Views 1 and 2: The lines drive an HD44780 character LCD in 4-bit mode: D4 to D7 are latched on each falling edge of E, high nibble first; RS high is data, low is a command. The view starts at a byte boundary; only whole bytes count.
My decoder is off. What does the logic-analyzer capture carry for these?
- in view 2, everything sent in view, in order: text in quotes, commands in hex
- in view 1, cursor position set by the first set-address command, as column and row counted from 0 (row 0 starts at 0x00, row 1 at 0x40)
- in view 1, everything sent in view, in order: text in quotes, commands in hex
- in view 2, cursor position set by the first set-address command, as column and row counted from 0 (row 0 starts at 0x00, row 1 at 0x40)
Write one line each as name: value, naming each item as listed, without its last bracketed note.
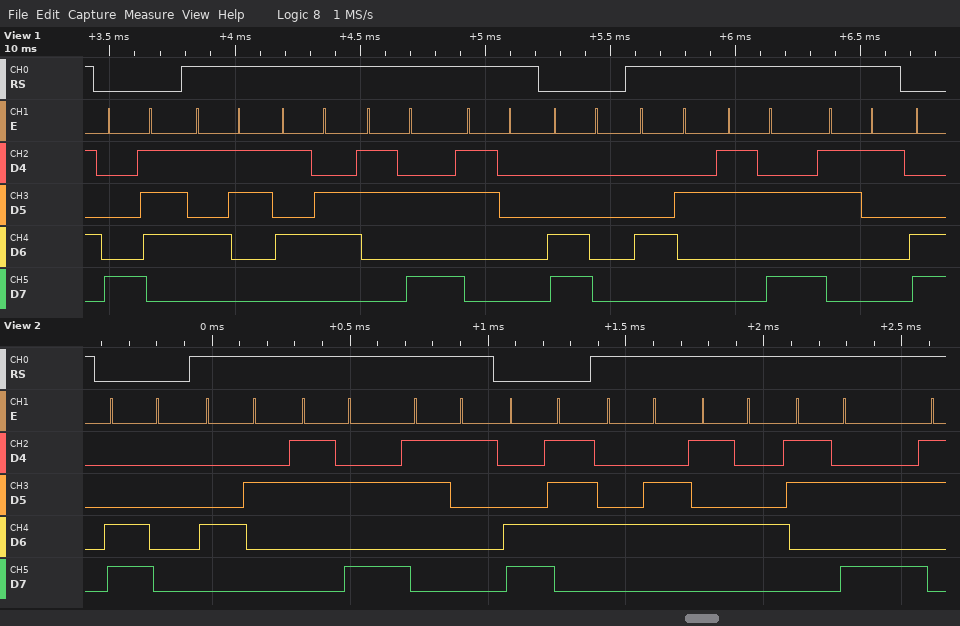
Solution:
in view 2, everything sent in view, in order: text in quotes, commands in hex: 0xC0 "B:1" 0xC7 "FT:"
in view 1, cursor position set by the first set-address command, as column and row counted from 0: column 7, row 0
in view 1, everything sent in view, in order: text in quotes, commands in hex: 0x87 "SV:0" 0xC0 "B:1"
in view 2, cursor position set by the first set-address command, as column and row counted from 0: column 0, row 1
